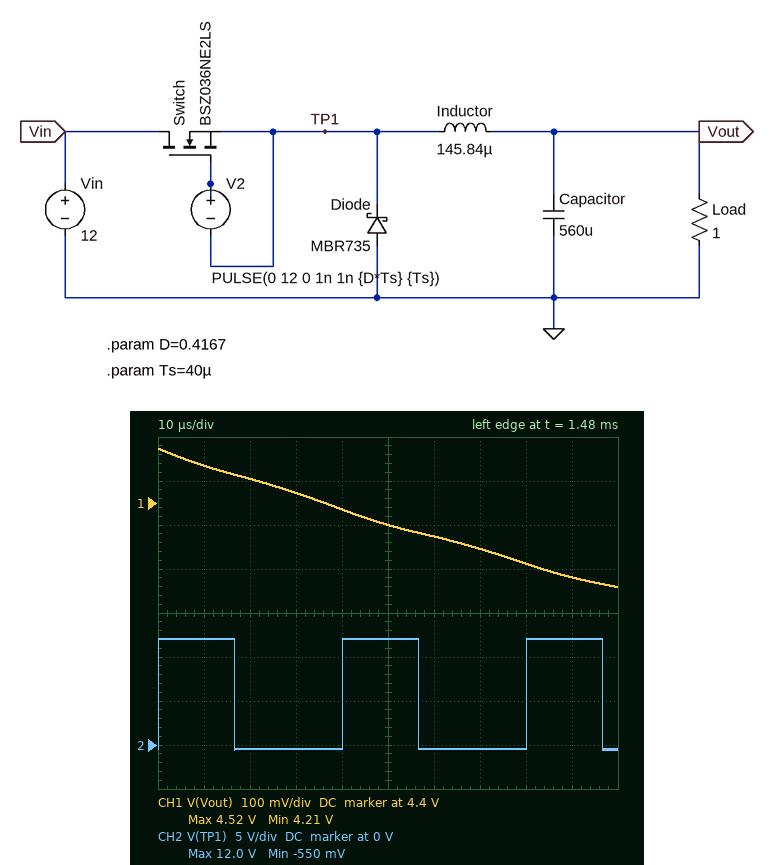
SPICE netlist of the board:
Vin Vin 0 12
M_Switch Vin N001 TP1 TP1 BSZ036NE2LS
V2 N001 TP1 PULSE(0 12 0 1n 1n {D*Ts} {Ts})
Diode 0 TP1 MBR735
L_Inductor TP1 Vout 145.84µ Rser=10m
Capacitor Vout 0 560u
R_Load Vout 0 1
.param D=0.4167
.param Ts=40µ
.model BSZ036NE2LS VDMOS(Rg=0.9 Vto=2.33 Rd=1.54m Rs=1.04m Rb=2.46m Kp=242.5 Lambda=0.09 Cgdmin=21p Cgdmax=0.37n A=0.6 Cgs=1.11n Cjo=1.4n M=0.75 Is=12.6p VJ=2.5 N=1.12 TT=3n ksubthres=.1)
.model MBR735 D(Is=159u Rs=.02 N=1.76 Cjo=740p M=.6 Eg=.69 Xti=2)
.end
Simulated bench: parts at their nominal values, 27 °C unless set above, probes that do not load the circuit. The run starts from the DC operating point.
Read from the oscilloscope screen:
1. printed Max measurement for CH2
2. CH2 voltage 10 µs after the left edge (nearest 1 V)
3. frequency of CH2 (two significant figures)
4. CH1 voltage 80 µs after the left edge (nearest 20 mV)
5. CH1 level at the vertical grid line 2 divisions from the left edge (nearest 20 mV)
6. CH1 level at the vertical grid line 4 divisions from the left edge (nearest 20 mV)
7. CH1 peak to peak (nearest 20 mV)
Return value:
12.0 V
12 V
25 kHz
4.26 V
4.46 V
4.38 V
320 mV
